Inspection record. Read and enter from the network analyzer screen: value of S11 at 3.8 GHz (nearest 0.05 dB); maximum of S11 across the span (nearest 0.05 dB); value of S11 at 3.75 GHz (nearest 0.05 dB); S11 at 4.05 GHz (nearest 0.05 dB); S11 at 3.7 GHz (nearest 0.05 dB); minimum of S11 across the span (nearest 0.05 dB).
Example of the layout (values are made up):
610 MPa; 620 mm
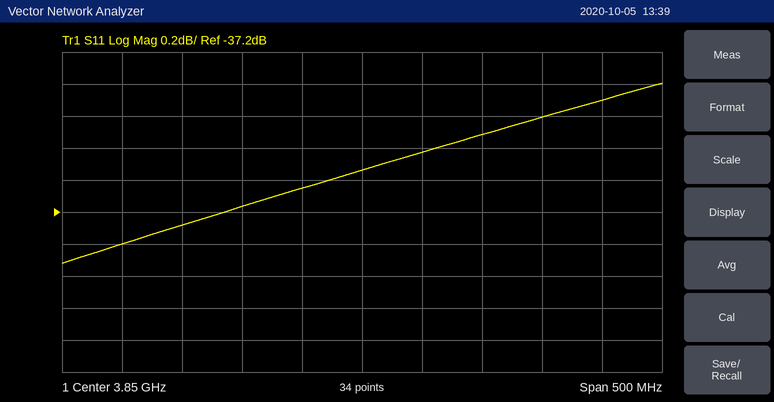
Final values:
-37.05 dB; -36.40 dB; -37.15 dB; -36.50 dB; -37.30 dB; -37.50 dB
